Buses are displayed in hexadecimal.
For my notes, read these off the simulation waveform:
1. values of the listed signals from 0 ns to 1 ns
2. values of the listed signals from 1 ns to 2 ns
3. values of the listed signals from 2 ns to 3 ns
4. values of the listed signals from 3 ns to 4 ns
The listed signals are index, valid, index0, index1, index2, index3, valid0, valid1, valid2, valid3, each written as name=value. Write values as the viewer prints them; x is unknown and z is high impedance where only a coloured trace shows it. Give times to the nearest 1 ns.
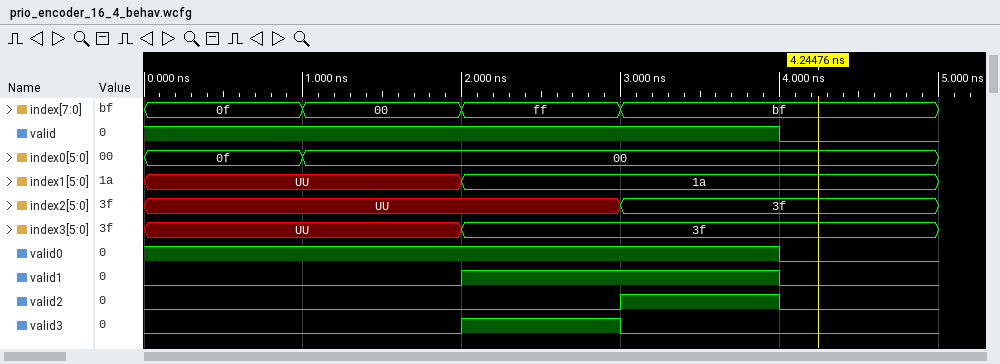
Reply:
index=0f, valid=1, index0=0f, index1=UU, index2=UU, index3=UU, valid0=1, valid1=0, valid2=0, valid3=0
index=00, valid=1, index0=00, index1=UU, index2=UU, index3=UU, valid0=1, valid1=0, valid2=0, valid3=0
index=ff, valid=1, index0=00, index1=1a, index2=UU, index3=3f, valid0=1, valid1=1, valid2=0, valid3=1
index=bf, valid=1, index0=00, index1=1a, index2=3f, index3=3f, valid0=1, valid1=1, valid2=1, valid3=0
